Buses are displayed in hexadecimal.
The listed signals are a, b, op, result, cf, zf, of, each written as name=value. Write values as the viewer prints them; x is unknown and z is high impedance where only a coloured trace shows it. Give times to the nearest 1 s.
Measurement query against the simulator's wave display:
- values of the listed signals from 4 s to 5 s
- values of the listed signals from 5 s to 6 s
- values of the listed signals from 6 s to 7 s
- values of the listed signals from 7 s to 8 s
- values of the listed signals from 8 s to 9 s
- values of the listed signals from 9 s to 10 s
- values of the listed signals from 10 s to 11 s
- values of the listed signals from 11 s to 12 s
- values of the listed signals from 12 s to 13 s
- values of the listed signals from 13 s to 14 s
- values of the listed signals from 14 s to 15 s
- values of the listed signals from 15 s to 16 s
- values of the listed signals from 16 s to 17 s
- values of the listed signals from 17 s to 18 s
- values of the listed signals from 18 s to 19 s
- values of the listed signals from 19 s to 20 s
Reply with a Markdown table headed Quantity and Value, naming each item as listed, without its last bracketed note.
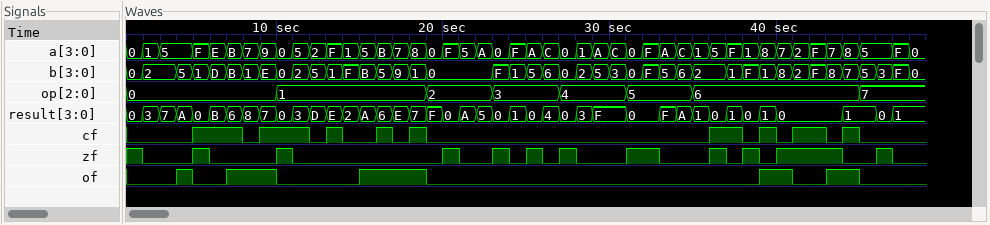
| Quantity | Value |
|---|---|
| values of the listed signals from 4 s to 5 s | a=5, b=5, op=0, result=A, cf=0, zf=0, of=1 |
| values of the listed signals from 5 s to 6 s | a=F, b=1, op=0, result=0, cf=1, zf=1, of=0 |
| values of the listed signals from 6 s to 7 s | a=E, b=D, op=0, result=B, cf=1, zf=0, of=0 |
| values of the listed signals from 7 s to 8 s | a=B, b=B, op=0, result=6, cf=1, zf=0, of=1 |
| values of the listed signals from 8 s to 9 s | a=7, b=1, op=0, result=8, cf=0, zf=0, of=1 |
| values of the listed signals from 9 s to 10 s | a=9, b=E, op=0, result=7, cf=1, zf=0, of=1 |
| values of the listed signals from 10 s to 11 s | a=0, b=0, op=1, result=0, cf=1, zf=1, of=0 |
| values of the listed signals from 11 s to 12 s | a=5, b=2, op=1, result=3, cf=1, zf=0, of=0 |
| values of the listed signals from 12 s to 13 s | a=2, b=5, op=1, result=D, cf=0, zf=0, of=0 |
| values of the listed signals from 13 s to 14 s | a=F, b=1, op=1, result=E, cf=1, zf=0, of=0 |
| values of the listed signals from 14 s to 15 s | a=1, b=F, op=1, result=2, cf=0, zf=0, of=0 |
| values of the listed signals from 15 s to 16 s | a=5, b=B, op=1, result=A, cf=0, zf=0, of=1 |
| values of the listed signals from 16 s to 17 s | a=B, b=5, op=1, result=6, cf=1, zf=0, of=1 |
| values of the listed signals from 17 s to 18 s | a=7, b=9, op=1, result=E, cf=0, zf=0, of=1 |
| values of the listed signals from 18 s to 19 s | a=8, b=1, op=1, result=7, cf=1, zf=0, of=1 |
| values of the listed signals from 19 s to 20 s | a=0, b=0, op=2, result=F, cf=0, zf=0, of=0 |
